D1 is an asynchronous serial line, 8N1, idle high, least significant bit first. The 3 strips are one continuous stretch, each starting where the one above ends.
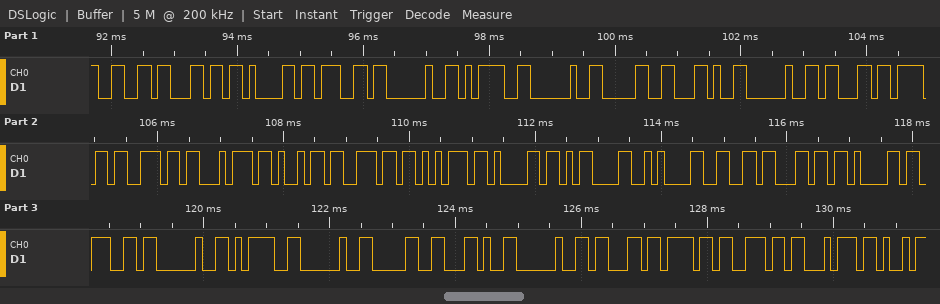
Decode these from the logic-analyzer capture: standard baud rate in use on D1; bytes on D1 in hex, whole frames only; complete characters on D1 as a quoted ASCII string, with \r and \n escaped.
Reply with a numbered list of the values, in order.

1. 9600 baud
2. 66 6C 61 67 20 3D 20 30 2C 20 63 6F 6E 74 69 6E 75 61 0D 0A 66 6C 61 67 20 3D 20 30 2C 20 63 6F 6E 74
3. "flag = 0, continua\r\nflag = 0, cont"
